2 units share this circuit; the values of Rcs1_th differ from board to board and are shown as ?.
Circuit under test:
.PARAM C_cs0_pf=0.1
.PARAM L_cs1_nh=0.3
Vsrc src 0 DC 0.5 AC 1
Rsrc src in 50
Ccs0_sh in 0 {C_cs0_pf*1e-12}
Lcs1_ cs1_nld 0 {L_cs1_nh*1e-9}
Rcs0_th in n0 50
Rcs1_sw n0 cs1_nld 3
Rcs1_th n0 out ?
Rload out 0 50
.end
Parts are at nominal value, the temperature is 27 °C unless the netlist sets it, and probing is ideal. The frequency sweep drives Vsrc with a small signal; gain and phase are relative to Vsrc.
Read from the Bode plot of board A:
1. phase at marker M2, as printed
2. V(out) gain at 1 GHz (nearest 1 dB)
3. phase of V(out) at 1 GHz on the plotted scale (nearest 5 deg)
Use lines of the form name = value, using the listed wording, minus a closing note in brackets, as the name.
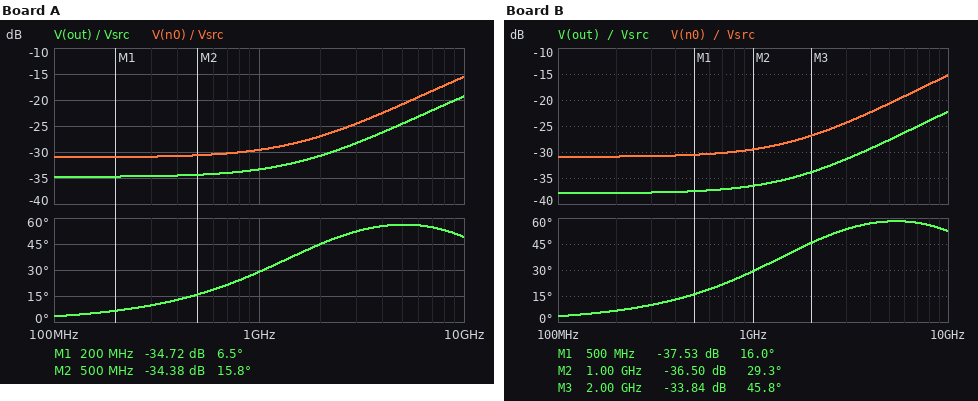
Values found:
phase at marker M2, as printed = 15.8 deg
V(out) gain at 1 GHz = -33 dB
phase of V(out) at 1 GHz on the plotted scale = 30 deg
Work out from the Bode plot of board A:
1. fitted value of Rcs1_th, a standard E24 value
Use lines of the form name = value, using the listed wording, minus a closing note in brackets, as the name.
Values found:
fitted value of Rcs1_th, a standard E24 value = 27 Ω
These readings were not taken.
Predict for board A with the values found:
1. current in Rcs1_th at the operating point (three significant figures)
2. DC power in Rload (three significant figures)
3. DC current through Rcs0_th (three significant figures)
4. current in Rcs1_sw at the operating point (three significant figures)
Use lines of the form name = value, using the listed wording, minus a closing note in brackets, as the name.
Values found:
current in Rcs1_th at the operating point = 182 µA
DC power in Rload = 1.66 µW
DC current through Rcs0_th = 4.86 mA
current in Rcs1_sw at the operating point = 4.68 mA
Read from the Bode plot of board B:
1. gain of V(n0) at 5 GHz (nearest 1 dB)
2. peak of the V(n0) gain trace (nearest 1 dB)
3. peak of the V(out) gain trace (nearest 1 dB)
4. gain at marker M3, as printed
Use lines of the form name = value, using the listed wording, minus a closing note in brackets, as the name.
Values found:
gain of V(n0) at 5 GHz = -21 dB
peak of the V(n0) gain trace = -15 dB
peak of the V(out) gain trace = -22 dB
gain at marker M3, as printed = -33.84 dB
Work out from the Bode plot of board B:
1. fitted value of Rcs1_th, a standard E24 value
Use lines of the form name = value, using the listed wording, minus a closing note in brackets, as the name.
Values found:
fitted value of Rcs1_th, a standard E24 value = 62 Ω
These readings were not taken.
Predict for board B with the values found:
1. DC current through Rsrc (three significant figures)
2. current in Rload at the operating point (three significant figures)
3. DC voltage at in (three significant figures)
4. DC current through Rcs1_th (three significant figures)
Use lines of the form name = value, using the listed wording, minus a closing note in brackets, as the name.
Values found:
DC current through Rsrc = 4.86 mA
current in Rload at the operating point = 127 µA
DC voltage at in = 257 mV
DC current through Rcs1_th = 127 µA
